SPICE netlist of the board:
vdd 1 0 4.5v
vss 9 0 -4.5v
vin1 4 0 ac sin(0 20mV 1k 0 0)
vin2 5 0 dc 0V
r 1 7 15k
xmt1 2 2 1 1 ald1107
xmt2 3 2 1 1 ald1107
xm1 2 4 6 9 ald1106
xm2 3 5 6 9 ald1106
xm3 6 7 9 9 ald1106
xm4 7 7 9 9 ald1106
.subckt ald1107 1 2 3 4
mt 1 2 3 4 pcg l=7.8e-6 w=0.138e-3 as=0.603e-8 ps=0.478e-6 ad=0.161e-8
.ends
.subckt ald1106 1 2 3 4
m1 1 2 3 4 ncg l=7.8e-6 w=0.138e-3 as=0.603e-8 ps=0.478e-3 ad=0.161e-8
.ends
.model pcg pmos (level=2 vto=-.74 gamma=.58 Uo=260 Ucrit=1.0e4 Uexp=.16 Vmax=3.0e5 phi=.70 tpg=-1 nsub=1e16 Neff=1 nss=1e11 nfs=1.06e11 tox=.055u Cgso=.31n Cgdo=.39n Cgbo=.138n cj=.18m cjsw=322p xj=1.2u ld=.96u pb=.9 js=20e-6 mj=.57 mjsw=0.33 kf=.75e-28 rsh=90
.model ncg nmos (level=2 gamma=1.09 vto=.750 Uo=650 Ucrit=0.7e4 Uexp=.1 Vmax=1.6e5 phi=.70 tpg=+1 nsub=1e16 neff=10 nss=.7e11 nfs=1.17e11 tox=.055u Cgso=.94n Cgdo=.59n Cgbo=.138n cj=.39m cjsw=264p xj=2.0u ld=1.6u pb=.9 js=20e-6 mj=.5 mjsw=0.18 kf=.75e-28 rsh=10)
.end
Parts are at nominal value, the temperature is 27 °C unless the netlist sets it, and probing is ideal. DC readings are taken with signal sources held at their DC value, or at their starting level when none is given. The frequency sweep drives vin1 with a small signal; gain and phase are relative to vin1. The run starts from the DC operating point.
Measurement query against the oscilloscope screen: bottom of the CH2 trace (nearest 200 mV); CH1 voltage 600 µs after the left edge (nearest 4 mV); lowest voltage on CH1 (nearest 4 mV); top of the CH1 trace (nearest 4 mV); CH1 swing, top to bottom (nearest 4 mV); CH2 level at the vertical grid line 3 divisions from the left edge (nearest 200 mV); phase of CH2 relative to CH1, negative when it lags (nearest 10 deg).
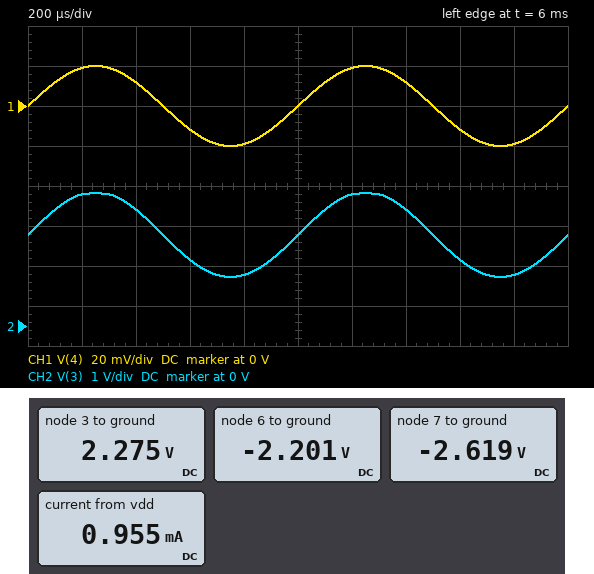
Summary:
1.2 V
-12 mV
-20 mV
20 mV
40 mV
1.6 V
0 deg
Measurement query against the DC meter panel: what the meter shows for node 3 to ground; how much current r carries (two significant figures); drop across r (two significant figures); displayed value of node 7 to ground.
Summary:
2.275 V
470 µA
7.1 V
-2.619 V
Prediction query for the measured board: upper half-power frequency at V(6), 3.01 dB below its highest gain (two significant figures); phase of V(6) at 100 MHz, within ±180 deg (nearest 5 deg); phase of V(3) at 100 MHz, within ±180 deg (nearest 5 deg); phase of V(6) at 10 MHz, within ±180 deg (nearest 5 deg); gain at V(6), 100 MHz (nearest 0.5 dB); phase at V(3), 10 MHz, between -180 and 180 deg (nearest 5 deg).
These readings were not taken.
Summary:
5.5 MHz
-35 deg
-140 deg
-20 deg
-13.0 dB
-80 deg
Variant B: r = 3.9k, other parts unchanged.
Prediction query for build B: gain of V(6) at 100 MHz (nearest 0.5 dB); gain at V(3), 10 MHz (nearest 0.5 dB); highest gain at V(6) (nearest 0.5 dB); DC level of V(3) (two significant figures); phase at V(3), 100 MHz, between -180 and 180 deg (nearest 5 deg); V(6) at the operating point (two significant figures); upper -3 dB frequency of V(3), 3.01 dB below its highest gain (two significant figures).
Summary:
-11.5 dB
27.5 dB
-4.0 dB
960 mV
-125 deg
-2.7 V
7.7 MHz
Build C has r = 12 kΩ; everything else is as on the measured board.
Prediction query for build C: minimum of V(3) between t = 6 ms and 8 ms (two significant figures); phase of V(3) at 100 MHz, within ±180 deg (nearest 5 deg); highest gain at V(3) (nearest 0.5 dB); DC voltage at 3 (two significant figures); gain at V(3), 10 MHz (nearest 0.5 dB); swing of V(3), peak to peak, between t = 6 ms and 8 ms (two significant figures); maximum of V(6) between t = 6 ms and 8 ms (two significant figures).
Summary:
1.1 V
-135 deg
34.0 dB
2.1 V
25.0 dB
2.0 V
-2.3 V
